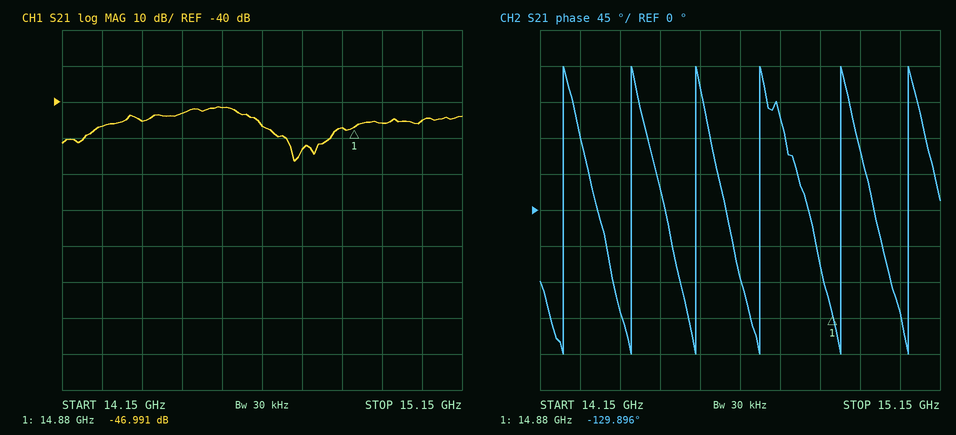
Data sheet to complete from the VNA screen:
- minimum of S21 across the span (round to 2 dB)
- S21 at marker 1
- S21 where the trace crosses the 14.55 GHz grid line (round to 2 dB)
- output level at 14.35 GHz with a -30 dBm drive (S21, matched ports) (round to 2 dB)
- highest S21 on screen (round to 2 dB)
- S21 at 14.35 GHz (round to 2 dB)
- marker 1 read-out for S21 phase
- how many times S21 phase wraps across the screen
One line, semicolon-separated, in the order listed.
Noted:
-56 dB; -46.991 dB; -42 dB; -76 dBm; -42 dB; -46 dB; -129.896°; 6
